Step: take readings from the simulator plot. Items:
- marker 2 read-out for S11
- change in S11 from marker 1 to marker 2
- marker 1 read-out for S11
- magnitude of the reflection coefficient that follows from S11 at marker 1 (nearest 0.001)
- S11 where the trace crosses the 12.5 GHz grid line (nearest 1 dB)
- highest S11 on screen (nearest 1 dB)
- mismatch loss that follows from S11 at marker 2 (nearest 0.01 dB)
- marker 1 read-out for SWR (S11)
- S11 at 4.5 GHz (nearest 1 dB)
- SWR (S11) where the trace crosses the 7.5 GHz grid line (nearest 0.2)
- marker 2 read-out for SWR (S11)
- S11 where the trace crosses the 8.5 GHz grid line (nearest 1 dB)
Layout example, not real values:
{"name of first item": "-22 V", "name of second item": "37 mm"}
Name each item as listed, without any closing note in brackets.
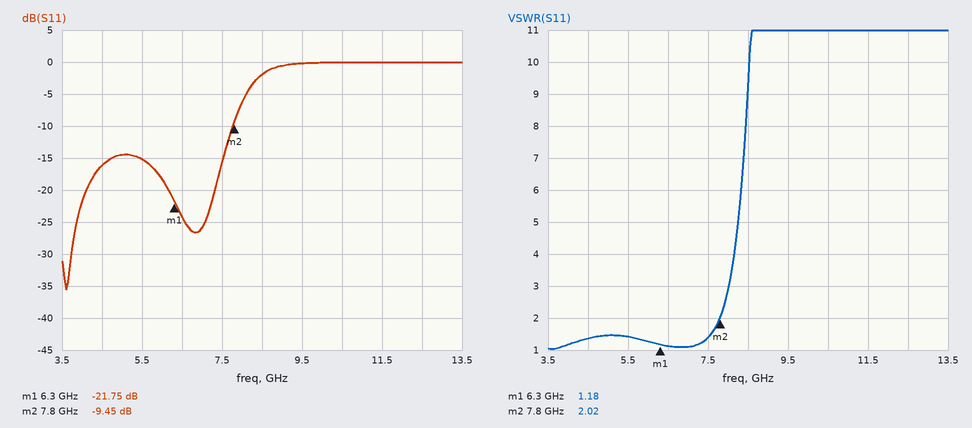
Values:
{"marker 2 read-out for S11": "-9.45 dB", "change in S11 from marker 1 to marker 2": "12.30 dB", "marker 1 read-out for S11": "-21.75 dB", "magnitude of the reflection coefficient that follows from S11 at marker 1": "0.082", "S11 where the trace crosses the 12.5 GHz grid line": "0 dB", "highest S11 on screen": "0 dB", "mismatch loss that follows from S11 at marker 2": "0.52 dB", "marker 1 read-out for SWR": "1.18", "S11 at 4.5 GHz": "-16 dB", "SWR (S11) where the trace crosses the 7.5 GHz grid line": "1.4", "marker 2 read-out for SWR": "2.02", "S11 where the trace crosses the 8.5 GHz grid line": "-2 dB"}
